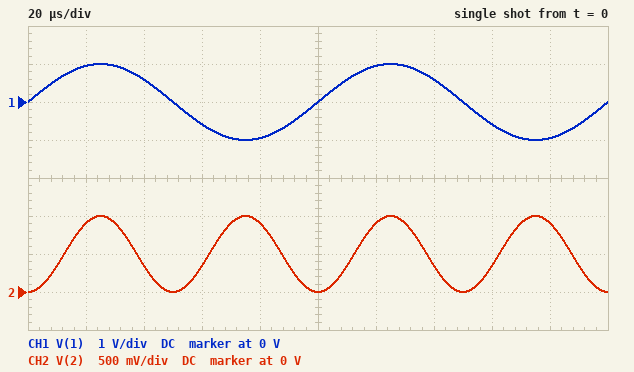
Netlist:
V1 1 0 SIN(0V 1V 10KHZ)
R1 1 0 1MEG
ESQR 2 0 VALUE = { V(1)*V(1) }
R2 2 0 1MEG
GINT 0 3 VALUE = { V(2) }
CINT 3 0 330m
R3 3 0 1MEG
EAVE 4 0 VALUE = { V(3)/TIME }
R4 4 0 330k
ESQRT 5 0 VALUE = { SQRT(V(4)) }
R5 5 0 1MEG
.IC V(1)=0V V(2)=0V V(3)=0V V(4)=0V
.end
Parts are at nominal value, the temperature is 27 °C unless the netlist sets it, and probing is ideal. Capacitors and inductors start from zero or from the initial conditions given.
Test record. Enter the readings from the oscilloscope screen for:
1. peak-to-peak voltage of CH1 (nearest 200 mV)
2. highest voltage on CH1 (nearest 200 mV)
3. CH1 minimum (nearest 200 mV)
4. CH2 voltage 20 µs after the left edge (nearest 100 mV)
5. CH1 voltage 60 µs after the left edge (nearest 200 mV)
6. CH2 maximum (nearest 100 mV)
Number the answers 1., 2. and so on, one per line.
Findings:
1. 2.0 V
2. 1.0 V
3. -1.0 V
4. 900 mV
5. -600 mV
6. 1.0 V
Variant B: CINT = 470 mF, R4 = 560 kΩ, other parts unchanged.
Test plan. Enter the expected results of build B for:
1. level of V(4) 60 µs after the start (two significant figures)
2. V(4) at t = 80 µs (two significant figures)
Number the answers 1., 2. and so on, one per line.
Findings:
1. 930 mV
2. 1.1 V
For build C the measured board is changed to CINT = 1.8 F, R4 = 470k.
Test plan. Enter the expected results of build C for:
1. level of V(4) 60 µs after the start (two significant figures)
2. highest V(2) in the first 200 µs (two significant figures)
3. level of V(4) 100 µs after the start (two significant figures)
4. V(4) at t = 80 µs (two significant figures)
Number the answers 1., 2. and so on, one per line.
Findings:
1. 240 mV
2. 1.0 V
3. 280 mV
4. 290 mV
